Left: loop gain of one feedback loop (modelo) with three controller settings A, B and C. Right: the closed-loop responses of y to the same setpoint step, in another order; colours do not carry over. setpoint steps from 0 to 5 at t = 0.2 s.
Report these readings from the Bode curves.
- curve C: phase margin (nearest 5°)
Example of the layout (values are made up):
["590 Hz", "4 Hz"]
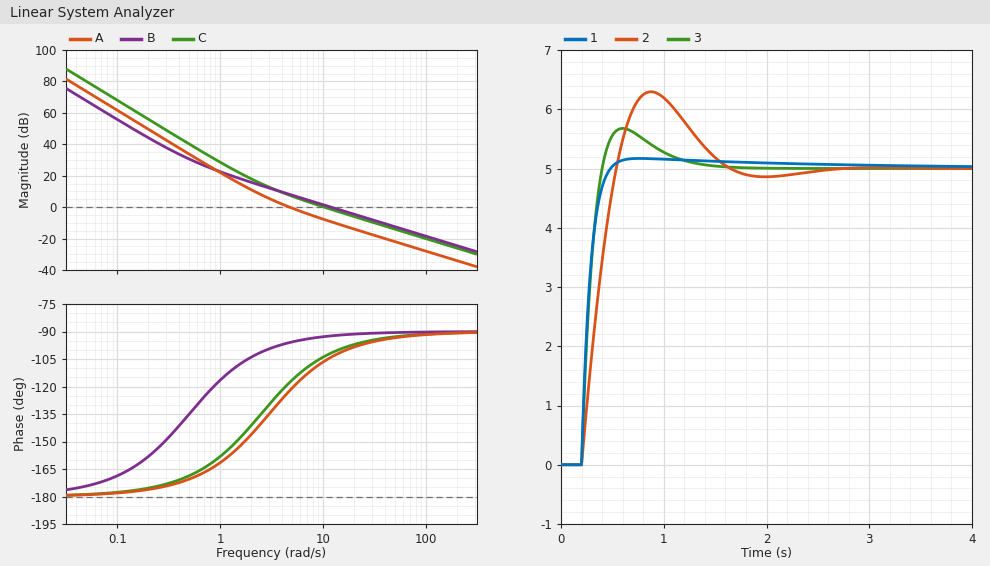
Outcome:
["75°"]
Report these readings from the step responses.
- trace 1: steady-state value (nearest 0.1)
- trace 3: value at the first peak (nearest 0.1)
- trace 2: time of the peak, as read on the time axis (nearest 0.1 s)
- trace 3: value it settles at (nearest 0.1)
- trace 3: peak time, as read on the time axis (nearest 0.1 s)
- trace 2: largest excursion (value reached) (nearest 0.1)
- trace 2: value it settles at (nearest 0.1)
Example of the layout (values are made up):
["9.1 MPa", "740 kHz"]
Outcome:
["5.0", "5.7", "0.9 s", "5.0", "0.6 s", "6.3", "5.0"]
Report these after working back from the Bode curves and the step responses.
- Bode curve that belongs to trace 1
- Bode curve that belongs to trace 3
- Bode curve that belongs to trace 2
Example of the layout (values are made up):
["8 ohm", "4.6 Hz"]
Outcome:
["B", "C", "A"]
